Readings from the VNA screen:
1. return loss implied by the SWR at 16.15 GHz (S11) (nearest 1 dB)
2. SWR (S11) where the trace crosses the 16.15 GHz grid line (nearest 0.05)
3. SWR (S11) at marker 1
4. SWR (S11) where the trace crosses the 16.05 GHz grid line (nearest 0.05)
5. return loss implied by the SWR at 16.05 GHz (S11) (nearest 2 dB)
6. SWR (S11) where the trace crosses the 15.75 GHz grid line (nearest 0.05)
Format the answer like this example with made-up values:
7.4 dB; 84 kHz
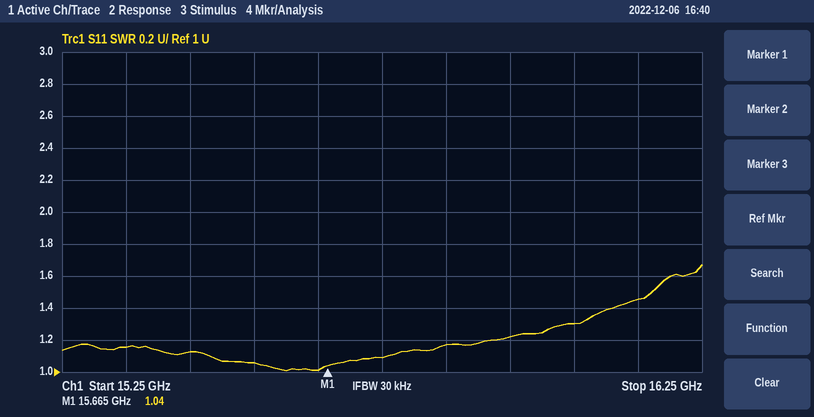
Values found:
15 dB; 1.45; 1.04; 1.30; 18 dB; 1.10
